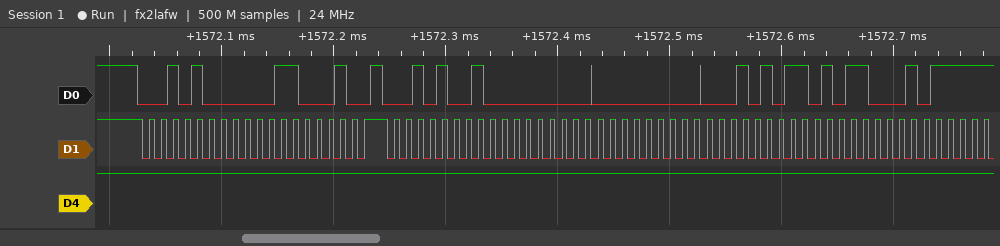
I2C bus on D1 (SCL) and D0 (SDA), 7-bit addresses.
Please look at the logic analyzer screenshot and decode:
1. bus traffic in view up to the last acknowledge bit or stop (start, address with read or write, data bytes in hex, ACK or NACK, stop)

start, address 14 write ACK, 31 ACK, stop, start, address 14 read ACK, 00 ACK, 00 ACK, 2B ACK, B1 ACK
